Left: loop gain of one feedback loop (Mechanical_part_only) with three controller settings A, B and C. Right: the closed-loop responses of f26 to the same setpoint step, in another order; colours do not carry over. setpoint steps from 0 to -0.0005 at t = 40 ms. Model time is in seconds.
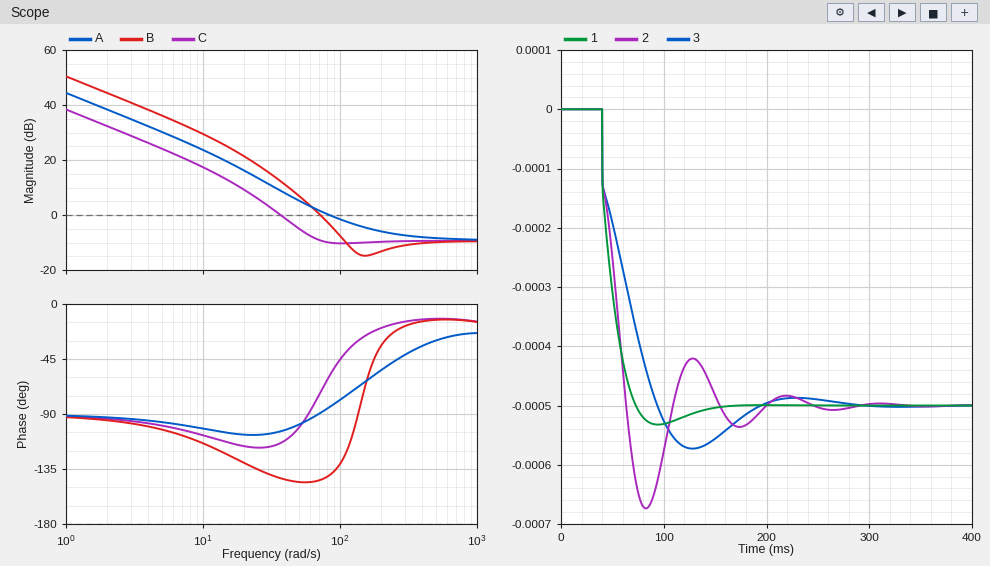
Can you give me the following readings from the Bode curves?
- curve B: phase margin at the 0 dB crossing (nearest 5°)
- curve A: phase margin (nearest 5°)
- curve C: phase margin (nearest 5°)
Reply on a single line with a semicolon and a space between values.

35°; 95°; 65°
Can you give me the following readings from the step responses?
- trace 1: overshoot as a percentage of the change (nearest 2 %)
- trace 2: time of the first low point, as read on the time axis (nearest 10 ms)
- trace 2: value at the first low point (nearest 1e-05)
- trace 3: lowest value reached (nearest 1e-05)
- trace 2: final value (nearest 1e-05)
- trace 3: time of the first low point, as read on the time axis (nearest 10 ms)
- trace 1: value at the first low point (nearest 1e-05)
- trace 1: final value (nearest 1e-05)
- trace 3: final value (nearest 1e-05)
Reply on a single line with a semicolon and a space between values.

6 %; 80 ms; -0.00067; -0.00057; -0.00050; 130 ms; -0.00053; -0.00050; -0.00050
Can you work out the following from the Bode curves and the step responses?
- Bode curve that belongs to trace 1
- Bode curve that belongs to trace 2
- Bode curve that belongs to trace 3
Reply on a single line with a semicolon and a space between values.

A; B; C
